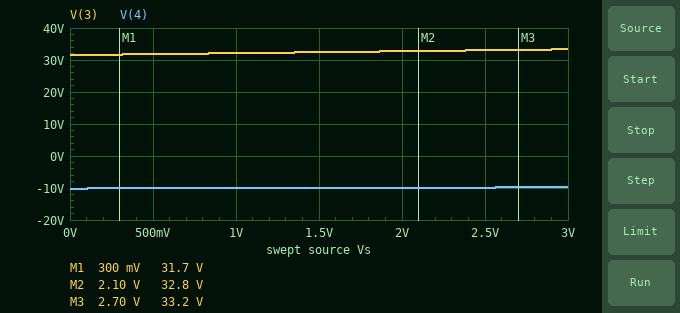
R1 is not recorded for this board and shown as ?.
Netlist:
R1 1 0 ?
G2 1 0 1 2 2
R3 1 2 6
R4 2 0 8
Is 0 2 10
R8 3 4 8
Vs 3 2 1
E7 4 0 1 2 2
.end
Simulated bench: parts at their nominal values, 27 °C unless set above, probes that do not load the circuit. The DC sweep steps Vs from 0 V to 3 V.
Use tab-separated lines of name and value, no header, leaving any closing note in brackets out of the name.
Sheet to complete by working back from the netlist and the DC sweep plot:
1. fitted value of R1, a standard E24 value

fitted value of R1, a standard E24 value	2.4 Ω
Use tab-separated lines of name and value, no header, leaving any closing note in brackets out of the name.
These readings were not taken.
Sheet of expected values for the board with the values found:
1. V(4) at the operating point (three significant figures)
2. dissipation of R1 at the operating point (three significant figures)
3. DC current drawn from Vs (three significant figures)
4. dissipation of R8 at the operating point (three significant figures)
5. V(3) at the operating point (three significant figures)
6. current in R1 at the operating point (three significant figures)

V(4) at the operating point	-10.0 V
dissipation of R1 at the operating point	284 W
DC current drawn from Vs	5.27 A
dissipation of R8 at the operating point	222 W
V(3) at the operating point	32.1 V
current in R1 at the operating point	10.9 A
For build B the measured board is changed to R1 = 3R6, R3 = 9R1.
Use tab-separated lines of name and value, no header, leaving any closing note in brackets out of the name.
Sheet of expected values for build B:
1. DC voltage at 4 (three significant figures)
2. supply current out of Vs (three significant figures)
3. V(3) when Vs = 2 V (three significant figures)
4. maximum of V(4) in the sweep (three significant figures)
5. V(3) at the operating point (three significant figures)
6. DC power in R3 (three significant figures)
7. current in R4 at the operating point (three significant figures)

DC voltage at 4	-7.87 V
supply current out of Vs	5.34 A
V(3) when Vs = 2 V	35.4 V
maximum of V(4) in the sweep	-7.67 V
V(3) at the operating point	34.8 V
DC power in R3	1.70 W
current in R4 at the operating point	4.23 A
